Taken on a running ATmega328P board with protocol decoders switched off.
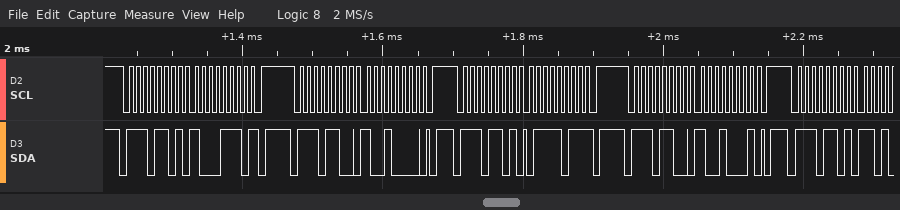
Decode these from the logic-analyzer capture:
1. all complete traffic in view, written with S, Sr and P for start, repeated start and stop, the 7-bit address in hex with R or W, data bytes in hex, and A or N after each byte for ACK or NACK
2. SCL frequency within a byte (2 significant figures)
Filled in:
S 76R A 8E N P S 76W A 90 A P S 76R A 7B N P S 76W A 91 A P S 76R A
100 kHz
